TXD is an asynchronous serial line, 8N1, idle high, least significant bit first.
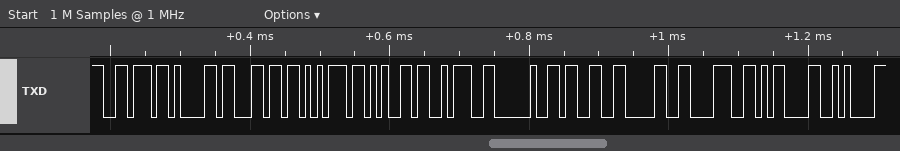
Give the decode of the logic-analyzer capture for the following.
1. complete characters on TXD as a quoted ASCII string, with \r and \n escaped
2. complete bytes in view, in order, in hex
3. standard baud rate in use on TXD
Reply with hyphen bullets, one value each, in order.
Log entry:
- "value: 308\r\n"
- 0x76 0x61 0x6C 0x75 0x65 0x3A 0x20 0x33 0x30 0x38 0x0D 0x0A
- 115200 baud
